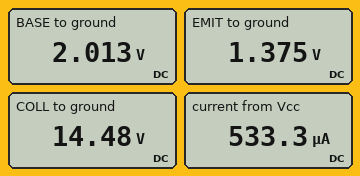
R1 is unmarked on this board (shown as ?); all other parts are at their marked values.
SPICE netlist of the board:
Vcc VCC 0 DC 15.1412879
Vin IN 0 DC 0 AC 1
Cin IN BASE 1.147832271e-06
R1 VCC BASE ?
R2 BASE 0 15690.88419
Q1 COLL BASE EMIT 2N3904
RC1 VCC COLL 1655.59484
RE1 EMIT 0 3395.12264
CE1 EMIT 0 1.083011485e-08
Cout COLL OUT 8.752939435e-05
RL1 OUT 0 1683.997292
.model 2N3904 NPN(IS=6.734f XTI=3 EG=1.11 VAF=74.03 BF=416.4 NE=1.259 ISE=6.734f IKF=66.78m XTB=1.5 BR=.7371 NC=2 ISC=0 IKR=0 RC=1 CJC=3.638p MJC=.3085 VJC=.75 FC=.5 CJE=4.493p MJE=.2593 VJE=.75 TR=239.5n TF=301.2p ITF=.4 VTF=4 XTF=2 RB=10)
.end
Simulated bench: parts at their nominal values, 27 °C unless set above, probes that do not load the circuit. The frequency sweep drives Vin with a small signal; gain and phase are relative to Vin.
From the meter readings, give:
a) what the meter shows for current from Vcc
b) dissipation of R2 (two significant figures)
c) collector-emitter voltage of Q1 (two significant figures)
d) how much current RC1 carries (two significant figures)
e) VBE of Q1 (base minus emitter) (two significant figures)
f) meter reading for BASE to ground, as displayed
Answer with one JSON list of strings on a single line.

["533.3 µA", "260 µW", "13 V", "400 µA", "640 mV", "2.013 V"]
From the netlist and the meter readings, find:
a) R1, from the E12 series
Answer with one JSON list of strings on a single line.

["100 kΩ"]
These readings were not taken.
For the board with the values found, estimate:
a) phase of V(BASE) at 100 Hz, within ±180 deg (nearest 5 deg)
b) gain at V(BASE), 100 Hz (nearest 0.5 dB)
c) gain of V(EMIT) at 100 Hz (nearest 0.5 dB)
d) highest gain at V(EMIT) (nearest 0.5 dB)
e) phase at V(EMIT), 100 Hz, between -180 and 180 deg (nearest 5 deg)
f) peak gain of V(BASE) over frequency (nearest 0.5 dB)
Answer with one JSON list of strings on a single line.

["5 deg", "0 dB", "0 dB", "0 dB", "5 deg", "0 dB"]
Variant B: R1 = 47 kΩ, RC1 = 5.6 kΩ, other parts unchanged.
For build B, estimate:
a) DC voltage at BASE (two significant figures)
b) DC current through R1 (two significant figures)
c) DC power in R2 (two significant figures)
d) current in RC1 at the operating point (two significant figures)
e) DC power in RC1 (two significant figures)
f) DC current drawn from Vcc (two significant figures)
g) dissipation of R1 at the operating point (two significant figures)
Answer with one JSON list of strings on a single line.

["3.7 V", "240 µA", "880 µW", "890 µA", "4.5 mW", "1.1 mA", "2.8 mW"]
